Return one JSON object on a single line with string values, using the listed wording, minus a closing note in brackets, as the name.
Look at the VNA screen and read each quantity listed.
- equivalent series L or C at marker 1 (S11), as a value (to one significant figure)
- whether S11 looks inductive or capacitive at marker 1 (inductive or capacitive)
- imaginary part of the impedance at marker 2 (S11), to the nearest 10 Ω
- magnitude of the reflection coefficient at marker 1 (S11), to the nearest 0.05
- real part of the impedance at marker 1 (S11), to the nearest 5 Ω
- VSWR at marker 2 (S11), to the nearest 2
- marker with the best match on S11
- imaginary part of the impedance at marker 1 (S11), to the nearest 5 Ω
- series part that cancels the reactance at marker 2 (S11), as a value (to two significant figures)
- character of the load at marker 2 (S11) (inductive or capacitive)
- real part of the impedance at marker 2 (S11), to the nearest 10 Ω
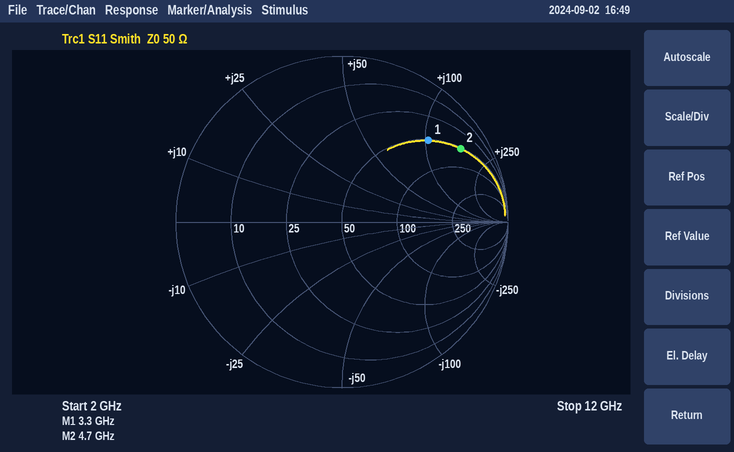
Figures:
{"equivalent series L or C at marker 1 (S11), as a value": "5 nH", "whether S11 looks inductive or capacitive at marker 1": "inductive", "imaginary part of the impedance at marker 2 (S11), to the nearest 10 Ω": "+160 Ω", "magnitude of the reflection coefficient at marker 1 (S11), to the nearest 0.05": "0.70", "real part of the impedance at marker 1 (S11), to the nearest 5 Ω": "50 Ω", "VSWR at marker 2 (S11), to the nearest 2": "12", "marker with the best match on S11": "marker 1", "imaginary part of the impedance at marker 1 (S11), to the nearest 5 Ω": "+105 Ω", "series part that cancels the reactance at marker 2 (S11), as a value": "210 fF", "character of the load at marker 2 (S11)": "inductive", "real part of the impedance at marker 2 (S11), to the nearest 10 Ω": "50 Ω"}
